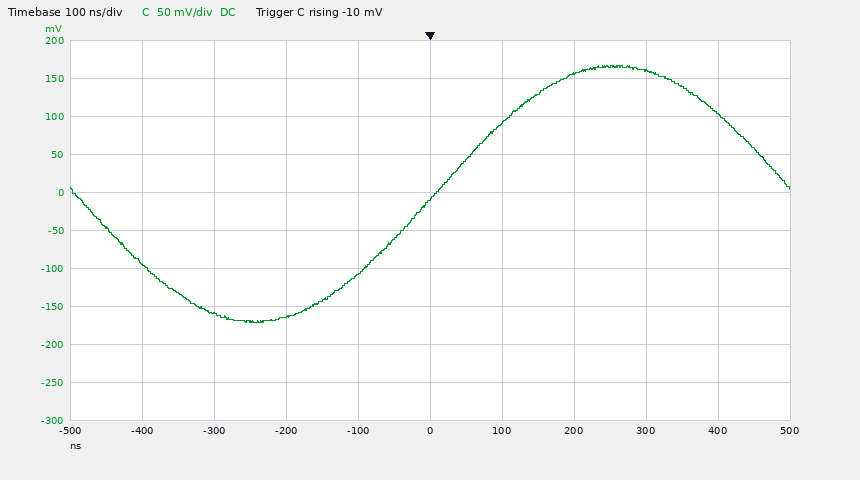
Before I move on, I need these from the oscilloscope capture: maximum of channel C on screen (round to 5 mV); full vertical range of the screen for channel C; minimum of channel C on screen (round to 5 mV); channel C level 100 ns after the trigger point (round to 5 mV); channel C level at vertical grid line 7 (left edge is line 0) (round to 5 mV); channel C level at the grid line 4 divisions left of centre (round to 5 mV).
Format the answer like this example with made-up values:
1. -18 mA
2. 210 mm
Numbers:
1. 165 mV
2. 500 mV
3. -170 mV
4. 90 mV
5. 155 mV
6. -95 mV
